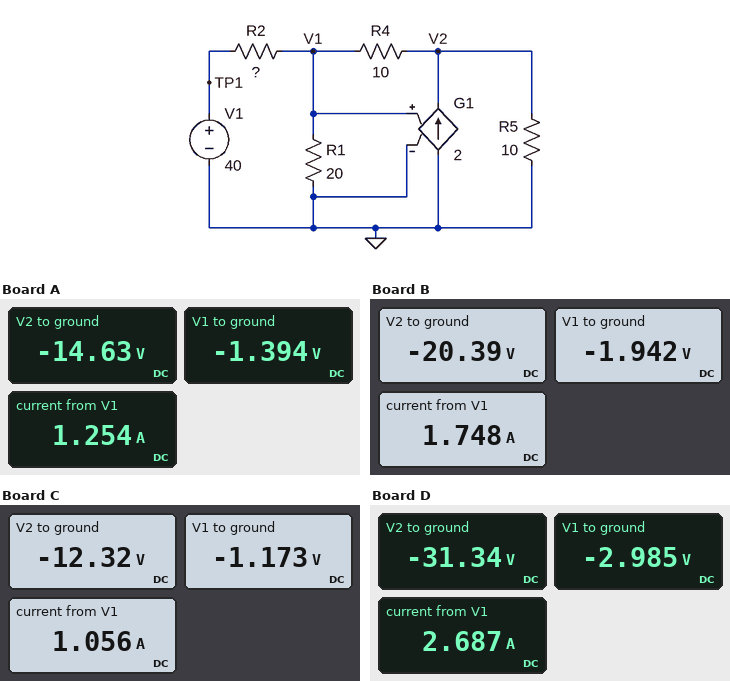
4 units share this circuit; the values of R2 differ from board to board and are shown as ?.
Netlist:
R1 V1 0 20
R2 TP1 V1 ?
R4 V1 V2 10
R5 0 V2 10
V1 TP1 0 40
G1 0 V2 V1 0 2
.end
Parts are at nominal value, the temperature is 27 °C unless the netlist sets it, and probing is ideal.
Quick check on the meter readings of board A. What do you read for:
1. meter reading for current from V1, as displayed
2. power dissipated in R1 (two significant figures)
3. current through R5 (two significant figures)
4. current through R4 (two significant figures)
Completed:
1.254 A
97 mW
1.5 A
1.3 A
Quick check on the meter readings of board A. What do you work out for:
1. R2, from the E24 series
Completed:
33 Ω
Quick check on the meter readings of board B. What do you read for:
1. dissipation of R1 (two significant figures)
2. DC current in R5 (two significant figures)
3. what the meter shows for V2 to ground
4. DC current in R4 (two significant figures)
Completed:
190 mW
2.0 A
-20.39 V
1.8 A
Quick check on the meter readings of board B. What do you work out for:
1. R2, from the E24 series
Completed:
24 Ω
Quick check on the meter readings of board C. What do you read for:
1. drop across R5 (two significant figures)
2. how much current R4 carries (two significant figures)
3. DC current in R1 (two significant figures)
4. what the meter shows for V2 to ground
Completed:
12 V
1.1 A
59 mA
-12.32 V
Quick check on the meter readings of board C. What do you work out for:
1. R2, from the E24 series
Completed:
39 Ω
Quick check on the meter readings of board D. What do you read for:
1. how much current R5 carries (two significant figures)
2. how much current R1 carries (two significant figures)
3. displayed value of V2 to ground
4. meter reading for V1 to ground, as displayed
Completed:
3.1 A
150 mA
-31.34 V
-2.985 V
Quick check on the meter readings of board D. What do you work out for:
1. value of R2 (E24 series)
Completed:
16 Ω
